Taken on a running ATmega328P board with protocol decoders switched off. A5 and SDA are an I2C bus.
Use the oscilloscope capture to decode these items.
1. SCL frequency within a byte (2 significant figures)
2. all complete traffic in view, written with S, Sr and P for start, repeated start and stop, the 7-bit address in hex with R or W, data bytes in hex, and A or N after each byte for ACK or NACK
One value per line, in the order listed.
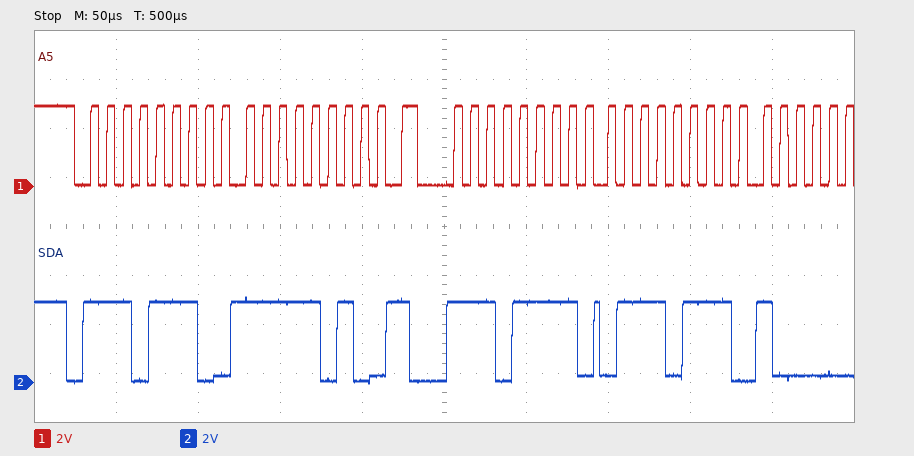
100 kHz
S 77W A FA A Sr 77R A 77 A
